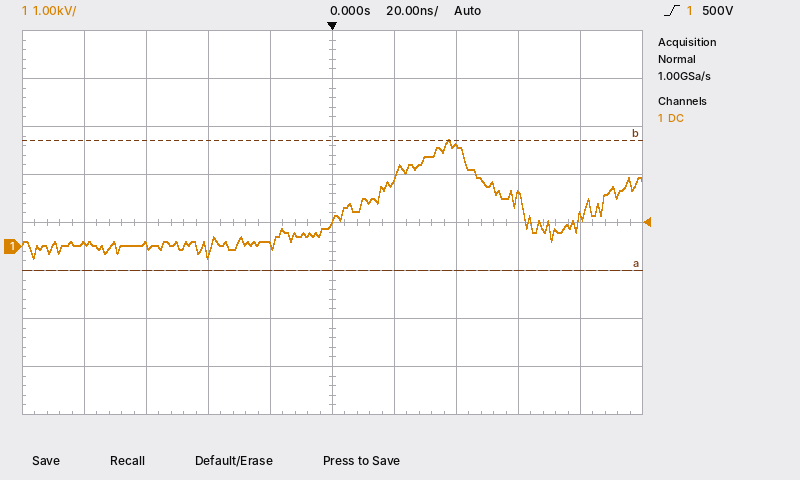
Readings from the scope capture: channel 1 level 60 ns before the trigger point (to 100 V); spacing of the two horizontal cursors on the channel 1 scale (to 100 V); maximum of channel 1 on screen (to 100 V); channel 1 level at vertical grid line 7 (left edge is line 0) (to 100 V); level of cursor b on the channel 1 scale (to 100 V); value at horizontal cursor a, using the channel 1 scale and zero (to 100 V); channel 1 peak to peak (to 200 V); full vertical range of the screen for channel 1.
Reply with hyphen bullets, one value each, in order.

- 0.0 kV
- 2.7 kV
- 2.2 kV
- 2.1 kV
- 2.2 kV
- -500 V
- 2.4 kV
- 8 kV
